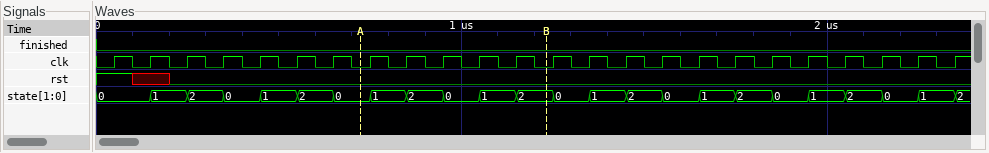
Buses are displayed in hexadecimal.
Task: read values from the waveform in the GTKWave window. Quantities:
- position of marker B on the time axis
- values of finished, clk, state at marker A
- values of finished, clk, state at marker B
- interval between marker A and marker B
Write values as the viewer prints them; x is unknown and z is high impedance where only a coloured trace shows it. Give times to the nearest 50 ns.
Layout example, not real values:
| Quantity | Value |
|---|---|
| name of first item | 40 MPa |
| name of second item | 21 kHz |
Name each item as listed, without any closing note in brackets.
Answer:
| Quantity | Value |
|---|---|
| position of marker B on the time axis | 1250 ns |
| values of finished, clk, state at marker A | finished=0, clk=0, state=0 |
| values of finished, clk, state at marker B | finished=0, clk=0, state=2 |
| interval between marker A and marker B | 500 ns |
